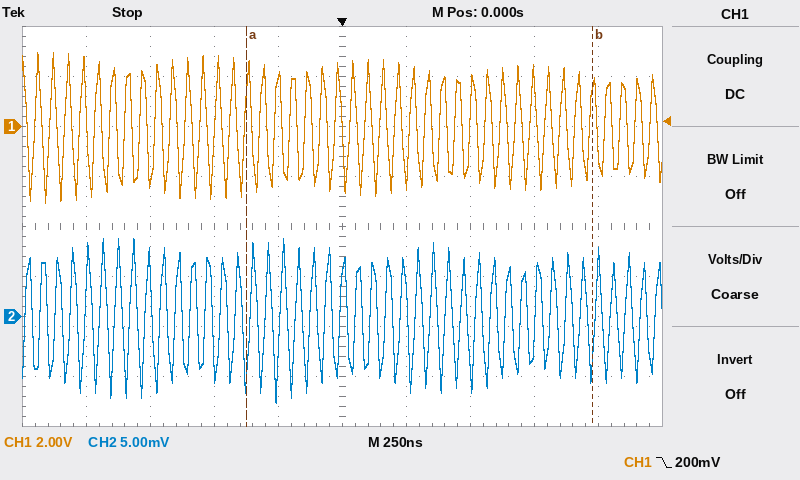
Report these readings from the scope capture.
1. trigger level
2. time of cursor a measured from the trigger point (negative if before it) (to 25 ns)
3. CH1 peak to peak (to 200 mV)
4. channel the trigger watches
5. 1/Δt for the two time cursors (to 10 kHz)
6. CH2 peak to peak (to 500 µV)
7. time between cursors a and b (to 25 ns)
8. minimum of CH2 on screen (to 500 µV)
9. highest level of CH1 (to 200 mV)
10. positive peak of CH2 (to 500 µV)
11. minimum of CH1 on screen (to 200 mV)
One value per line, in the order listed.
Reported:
200 mV
-375 ns
6.0 V
CH1
740 kHz
16.5 mV
1.350 µs
-8.5 mV
3.0 V
8.0 mV
-3.0 V
